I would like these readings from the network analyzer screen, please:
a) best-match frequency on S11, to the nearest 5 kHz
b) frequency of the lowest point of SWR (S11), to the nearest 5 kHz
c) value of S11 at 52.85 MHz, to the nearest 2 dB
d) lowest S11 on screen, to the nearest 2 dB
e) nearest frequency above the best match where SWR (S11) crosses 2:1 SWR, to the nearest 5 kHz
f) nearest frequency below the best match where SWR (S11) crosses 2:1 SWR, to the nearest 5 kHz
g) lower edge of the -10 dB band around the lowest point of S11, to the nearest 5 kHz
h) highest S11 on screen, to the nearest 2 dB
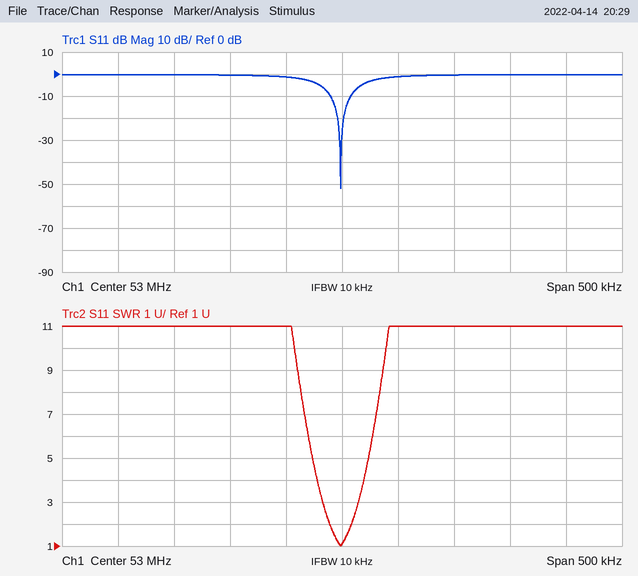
53.000 MHz
53.000 MHz
0 dB
-52 dB
53.010 MHz
52.990 MHz
52.990 MHz
0 dB
